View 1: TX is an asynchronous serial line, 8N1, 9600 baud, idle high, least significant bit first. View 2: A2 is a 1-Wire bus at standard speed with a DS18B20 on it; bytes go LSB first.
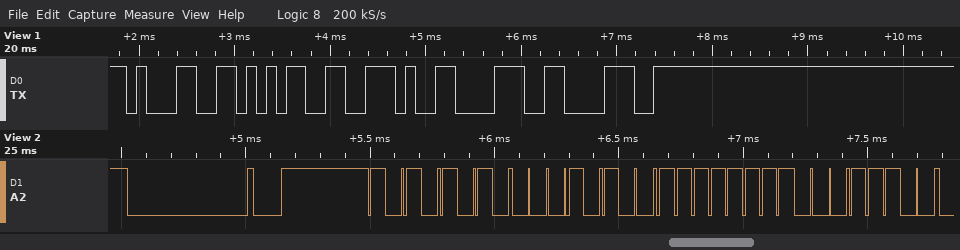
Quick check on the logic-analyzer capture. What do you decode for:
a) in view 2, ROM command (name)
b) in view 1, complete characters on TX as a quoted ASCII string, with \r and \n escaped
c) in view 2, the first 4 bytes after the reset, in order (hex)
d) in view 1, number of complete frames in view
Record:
Match ROM
"15.88"
55 28 FF 38
5
